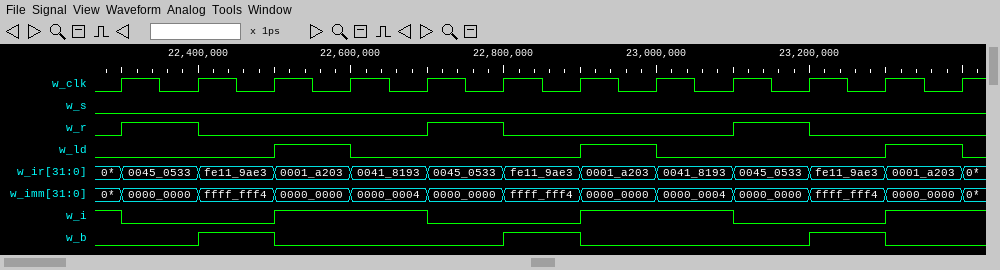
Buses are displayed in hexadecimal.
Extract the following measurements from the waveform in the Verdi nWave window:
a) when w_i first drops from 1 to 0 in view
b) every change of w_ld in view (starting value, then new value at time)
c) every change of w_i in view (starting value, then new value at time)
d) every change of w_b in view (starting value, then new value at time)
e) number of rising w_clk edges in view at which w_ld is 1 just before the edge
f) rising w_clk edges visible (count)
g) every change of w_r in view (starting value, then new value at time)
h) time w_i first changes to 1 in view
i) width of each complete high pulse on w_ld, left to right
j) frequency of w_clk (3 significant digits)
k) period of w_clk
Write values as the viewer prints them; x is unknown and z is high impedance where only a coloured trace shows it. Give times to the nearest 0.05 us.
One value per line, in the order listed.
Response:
22.3 us
0, 1 at 22.5 us, 0 at 22.6 us, 1 at 22.9 us, 0 at 23 us, 1 at 23.3 us, 0 at 23.4 us
1, 0 at 22.3 us, 1 at 22.5 us, 0 at 22.7 us, 1 at 22.9 us, 0 at 23.1 us, 1 at 23.3 us
0, 1 at 22.4 us, 0 at 22.5 us, 1 at 22.8 us, 0 at 22.9 us, 1 at 23.2 us, 0 at 23.3 us
3
12
0, 1 at 22.3 us, 0 at 22.4 us, 1 at 22.7 us, 0 at 22.8 us, 1 at 23.1 us, 0 at 23.2 us
22.5 us
0.1 us, 0.1 us, 0.1 us
10.0 MHz
0.1 us
